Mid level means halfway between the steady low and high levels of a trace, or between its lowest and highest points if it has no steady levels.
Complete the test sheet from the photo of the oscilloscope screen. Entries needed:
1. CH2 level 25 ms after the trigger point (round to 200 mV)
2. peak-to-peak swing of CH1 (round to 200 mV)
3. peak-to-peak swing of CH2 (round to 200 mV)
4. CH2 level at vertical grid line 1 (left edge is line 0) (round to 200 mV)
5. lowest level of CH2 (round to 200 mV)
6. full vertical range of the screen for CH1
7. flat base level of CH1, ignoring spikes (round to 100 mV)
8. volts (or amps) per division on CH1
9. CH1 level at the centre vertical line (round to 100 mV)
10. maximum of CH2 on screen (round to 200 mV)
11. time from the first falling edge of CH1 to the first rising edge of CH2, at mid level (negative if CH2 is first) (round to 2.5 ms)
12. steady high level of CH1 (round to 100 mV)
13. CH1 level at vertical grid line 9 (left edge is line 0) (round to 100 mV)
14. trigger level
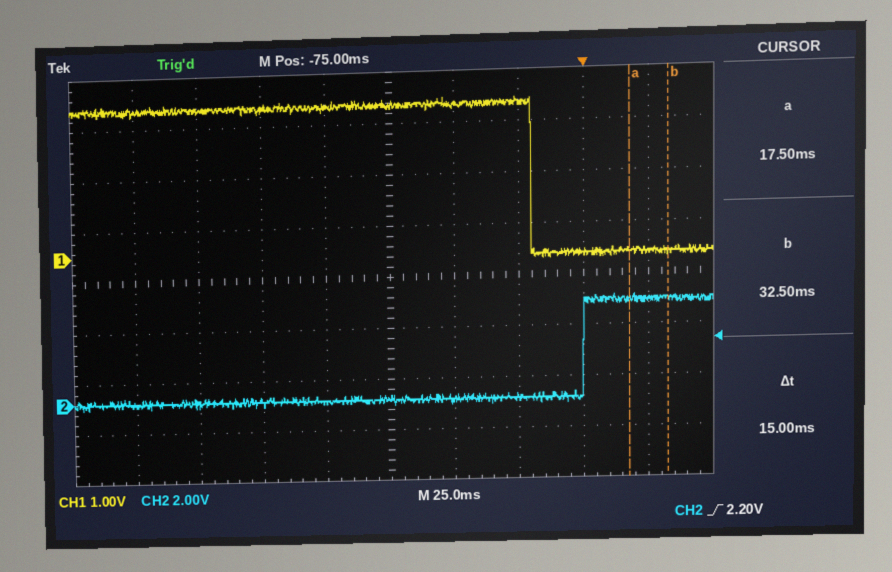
3.8 V
3.2 V
4.2 V
0.0 V
-200 mV
8 V
-100 mV
1 V
2.9 V
4.0 V
+20.0 ms
2.9 V
-100 mV
2.20 V
